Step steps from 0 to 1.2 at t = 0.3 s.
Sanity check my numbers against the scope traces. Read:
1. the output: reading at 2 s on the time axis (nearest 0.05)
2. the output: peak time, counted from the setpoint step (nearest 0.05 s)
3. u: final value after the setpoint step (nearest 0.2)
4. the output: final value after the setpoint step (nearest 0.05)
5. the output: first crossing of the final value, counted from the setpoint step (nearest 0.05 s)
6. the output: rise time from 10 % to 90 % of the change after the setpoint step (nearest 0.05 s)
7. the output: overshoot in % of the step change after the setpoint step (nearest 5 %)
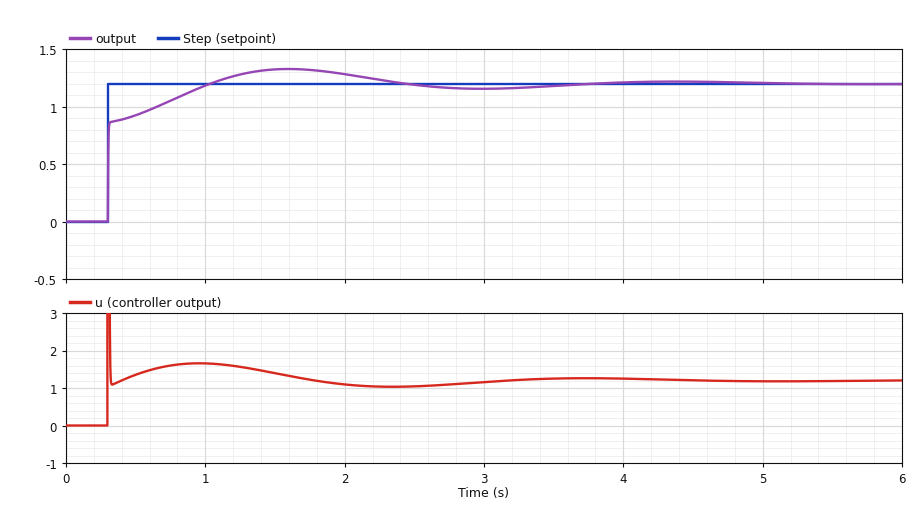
1.30
1.30 s
1.2
1.20
0.75 s
0.50 s
10 %
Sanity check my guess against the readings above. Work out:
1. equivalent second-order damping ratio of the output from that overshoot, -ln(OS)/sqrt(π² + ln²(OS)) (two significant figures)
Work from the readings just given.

0.59
